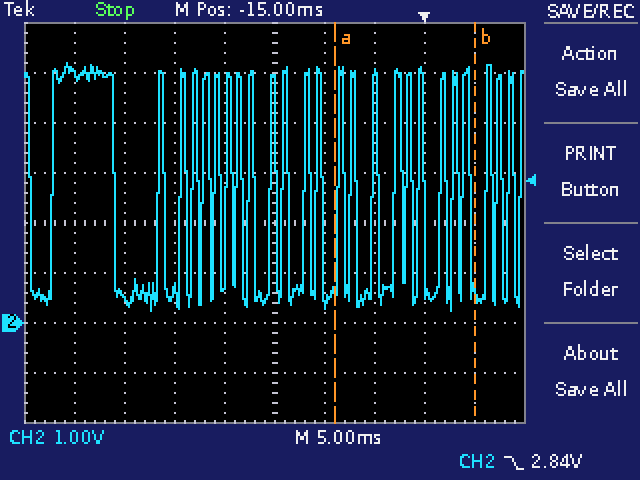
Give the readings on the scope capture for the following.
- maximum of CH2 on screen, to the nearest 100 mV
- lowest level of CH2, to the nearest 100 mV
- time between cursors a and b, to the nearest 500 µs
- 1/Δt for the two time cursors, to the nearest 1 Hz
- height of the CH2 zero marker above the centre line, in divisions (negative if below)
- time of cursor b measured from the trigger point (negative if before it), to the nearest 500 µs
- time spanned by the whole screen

5.2 V
200 mV
14.0 ms
71 Hz
-2.0 div
+5.0 ms
50 ms
